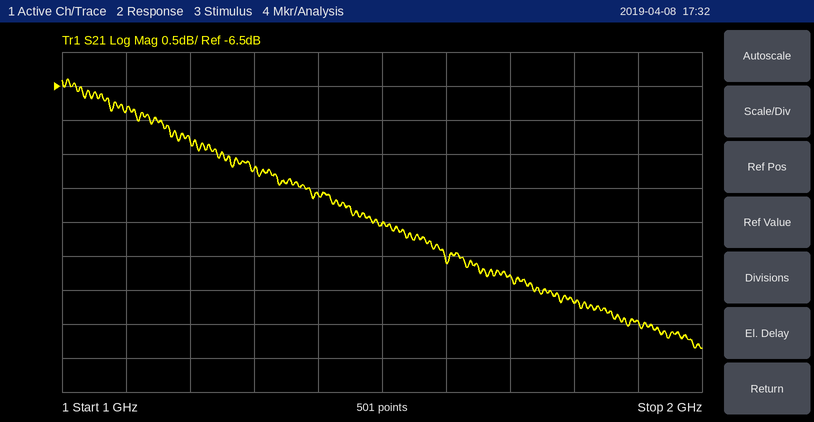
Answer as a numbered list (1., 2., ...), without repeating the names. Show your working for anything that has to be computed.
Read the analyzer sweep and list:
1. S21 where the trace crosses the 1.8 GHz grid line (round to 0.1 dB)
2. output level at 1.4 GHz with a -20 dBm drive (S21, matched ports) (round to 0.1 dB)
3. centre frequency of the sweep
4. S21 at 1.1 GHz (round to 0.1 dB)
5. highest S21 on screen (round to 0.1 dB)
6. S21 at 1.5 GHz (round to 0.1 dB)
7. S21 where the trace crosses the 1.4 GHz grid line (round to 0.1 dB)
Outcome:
1. -9.7 dB
2. -20 dBm + (-8.1 dB) = -28.1 dBm
3. 1.5 GHz
4. -6.9 dB
5. -6.4 dB
6. -8.5 dB
7. -8.1 dB
